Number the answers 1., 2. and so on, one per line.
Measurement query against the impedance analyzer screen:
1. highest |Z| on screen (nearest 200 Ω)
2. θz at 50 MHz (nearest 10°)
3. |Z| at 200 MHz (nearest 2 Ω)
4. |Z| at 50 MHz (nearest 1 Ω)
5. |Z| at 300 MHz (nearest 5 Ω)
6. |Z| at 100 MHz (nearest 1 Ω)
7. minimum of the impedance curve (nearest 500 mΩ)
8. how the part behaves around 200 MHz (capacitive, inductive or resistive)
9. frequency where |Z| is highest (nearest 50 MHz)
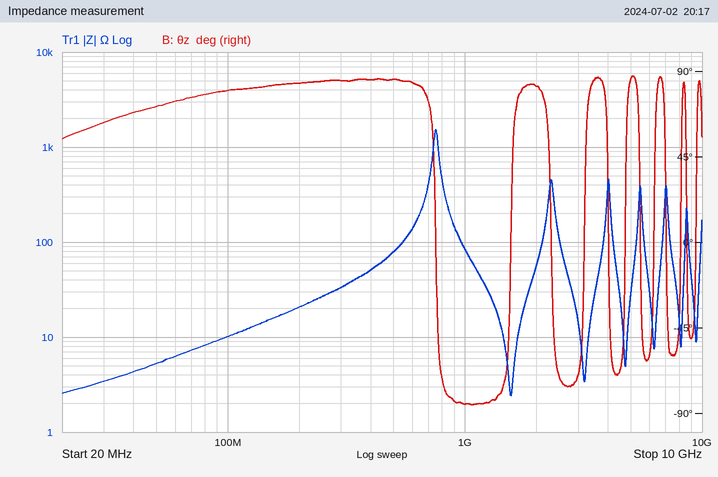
1. 1.6 kΩ
2. 70°
3. 20 Ω
4. 5 Ω
5. 35 Ω
6. 10 Ω
7. 2.5 Ω
8. inductive
9. 750 MHz
